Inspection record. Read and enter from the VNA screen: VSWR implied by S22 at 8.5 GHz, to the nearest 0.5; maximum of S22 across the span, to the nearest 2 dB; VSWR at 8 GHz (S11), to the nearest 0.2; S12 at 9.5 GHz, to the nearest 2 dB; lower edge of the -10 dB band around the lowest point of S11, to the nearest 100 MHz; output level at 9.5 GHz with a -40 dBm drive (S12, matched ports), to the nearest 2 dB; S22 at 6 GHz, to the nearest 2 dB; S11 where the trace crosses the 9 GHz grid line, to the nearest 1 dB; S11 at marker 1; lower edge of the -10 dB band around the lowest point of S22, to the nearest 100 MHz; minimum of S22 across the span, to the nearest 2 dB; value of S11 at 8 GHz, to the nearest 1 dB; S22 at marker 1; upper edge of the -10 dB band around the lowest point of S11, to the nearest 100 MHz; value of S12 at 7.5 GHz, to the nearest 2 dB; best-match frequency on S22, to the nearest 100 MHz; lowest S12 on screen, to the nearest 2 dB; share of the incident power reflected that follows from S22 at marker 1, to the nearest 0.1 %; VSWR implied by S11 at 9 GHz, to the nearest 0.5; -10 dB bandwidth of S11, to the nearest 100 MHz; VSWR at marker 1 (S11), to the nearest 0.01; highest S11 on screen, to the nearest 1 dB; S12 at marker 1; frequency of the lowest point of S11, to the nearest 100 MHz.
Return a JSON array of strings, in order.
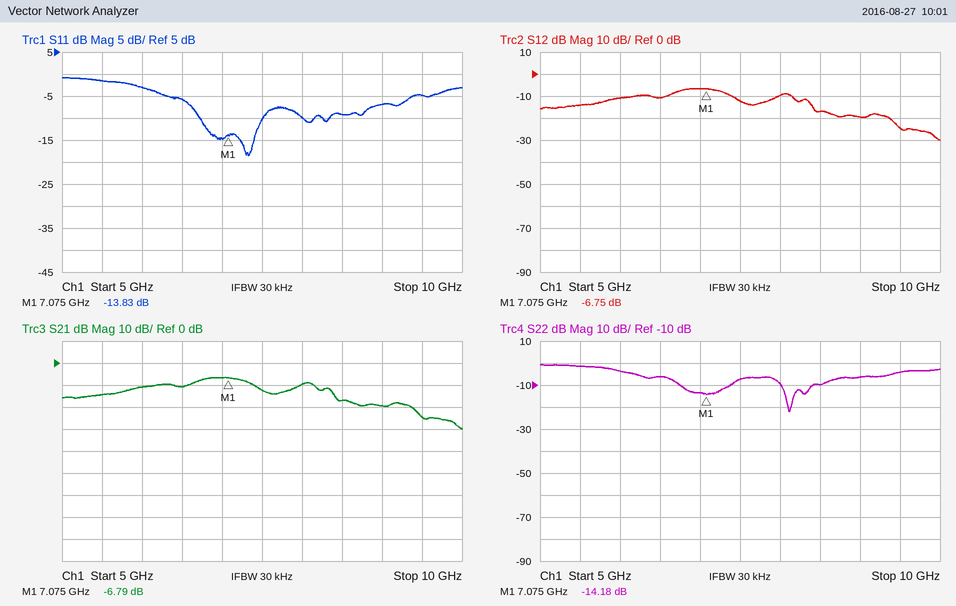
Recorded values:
["2.0", "0 dB", "2.0", "-24 dB", "6.7 GHz", "-64 dBm", "-4 dB", "-7 dB", "-13.83 dB", "8.0 GHz", "-22 dB", "-10 dB", "-14.18 dB", "7.5 GHz", "-12 dB", "8.1 GHz", "-30 dB", "3.8 %", "2.5", "800 MHz", "1.51", "-1 dB", "-6.75 dB", "7.3 GHz"]
